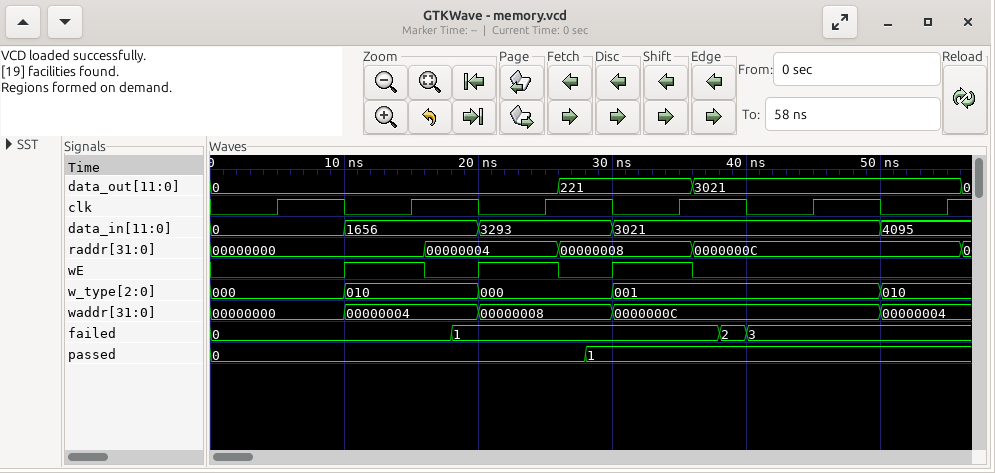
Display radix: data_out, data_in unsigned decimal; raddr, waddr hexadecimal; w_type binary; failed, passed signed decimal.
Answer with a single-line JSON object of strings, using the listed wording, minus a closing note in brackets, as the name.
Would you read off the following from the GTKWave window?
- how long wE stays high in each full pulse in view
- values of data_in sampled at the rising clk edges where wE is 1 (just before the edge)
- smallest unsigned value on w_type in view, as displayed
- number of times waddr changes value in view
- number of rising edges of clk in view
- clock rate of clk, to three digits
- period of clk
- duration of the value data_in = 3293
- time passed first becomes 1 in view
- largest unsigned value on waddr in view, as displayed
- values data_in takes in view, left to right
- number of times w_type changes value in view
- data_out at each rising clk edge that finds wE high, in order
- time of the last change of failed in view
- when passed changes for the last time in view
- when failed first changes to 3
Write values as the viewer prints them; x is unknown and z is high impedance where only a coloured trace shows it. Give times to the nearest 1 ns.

{"how long wE stays high in each full pulse in view": "6 ns, 6 ns, 6 ns", "values of data_in sampled at the rising clk edges where wE is 1": "1656, 3293, 3021", "smallest unsigned value on w_type in view, as displayed": "000", "number of times waddr changes value in view": "4", "number of rising edges of clk in view": "6", "clock rate of clk, to three digits": "100 MHz", "period of clk": "10 ns", "duration of the value data_in = 3293": "10 ns", "time passed first becomes 1 in view": "28 ns", "largest unsigned value on waddr in view, as displayed": "0000000C", "values data_in takes in view, left to right": "0, 1656, 3293, 3021, 4095", "number of times w_type changes value in view": "4", "data_out at each rising clk edge that finds wE high, in order": "0, 0, 221", "time of the last change of failed in view": "40 ns", "when passed changes for the last time in view": "28 ns", "when failed first changes to 3": "40 ns"}
